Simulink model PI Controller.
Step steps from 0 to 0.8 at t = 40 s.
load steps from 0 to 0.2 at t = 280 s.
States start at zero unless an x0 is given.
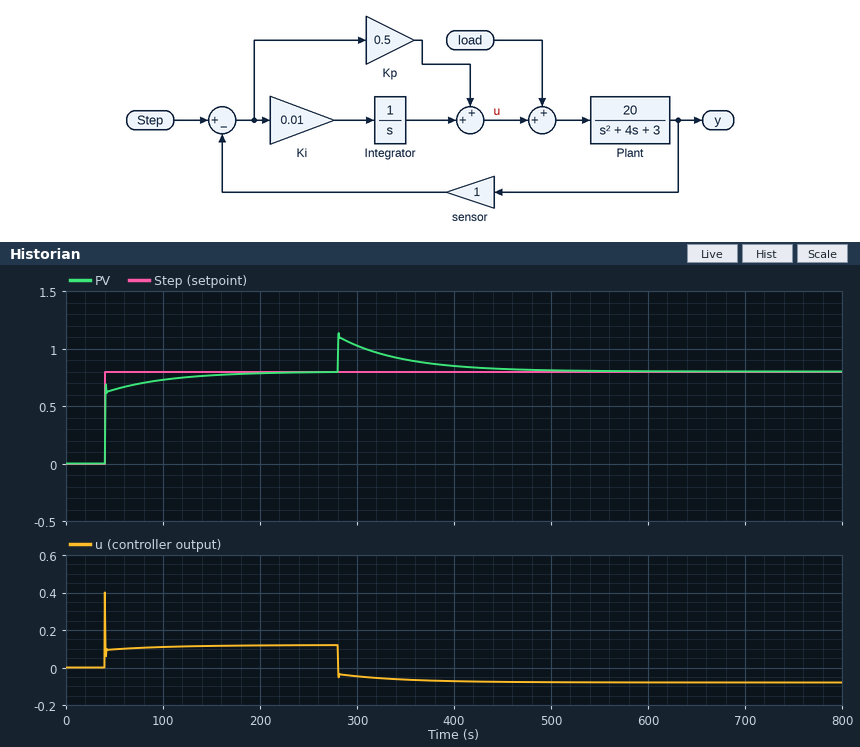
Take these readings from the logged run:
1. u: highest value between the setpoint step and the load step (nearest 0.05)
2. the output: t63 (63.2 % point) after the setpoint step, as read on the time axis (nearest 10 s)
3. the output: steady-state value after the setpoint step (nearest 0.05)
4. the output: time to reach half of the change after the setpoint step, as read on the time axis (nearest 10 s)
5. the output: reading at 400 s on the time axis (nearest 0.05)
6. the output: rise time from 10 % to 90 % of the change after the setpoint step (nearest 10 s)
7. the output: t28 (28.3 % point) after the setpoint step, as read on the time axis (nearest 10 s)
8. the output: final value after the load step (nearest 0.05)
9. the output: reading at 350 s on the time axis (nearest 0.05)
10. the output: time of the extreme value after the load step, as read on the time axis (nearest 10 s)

0.40
40 s
0.80
40 s
0.85
50 s
40 s
0.80
0.90
280 s
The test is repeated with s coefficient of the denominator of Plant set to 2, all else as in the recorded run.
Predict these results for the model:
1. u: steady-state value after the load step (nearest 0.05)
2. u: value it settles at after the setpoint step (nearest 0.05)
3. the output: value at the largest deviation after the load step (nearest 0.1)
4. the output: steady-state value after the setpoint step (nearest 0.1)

-0.10
0.10
1.2
0.8
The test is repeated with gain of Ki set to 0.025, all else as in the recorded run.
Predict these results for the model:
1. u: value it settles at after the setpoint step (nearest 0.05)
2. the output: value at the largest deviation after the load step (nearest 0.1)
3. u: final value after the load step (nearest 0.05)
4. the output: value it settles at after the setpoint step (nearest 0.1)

0.10
1.1
-0.10
0.8
